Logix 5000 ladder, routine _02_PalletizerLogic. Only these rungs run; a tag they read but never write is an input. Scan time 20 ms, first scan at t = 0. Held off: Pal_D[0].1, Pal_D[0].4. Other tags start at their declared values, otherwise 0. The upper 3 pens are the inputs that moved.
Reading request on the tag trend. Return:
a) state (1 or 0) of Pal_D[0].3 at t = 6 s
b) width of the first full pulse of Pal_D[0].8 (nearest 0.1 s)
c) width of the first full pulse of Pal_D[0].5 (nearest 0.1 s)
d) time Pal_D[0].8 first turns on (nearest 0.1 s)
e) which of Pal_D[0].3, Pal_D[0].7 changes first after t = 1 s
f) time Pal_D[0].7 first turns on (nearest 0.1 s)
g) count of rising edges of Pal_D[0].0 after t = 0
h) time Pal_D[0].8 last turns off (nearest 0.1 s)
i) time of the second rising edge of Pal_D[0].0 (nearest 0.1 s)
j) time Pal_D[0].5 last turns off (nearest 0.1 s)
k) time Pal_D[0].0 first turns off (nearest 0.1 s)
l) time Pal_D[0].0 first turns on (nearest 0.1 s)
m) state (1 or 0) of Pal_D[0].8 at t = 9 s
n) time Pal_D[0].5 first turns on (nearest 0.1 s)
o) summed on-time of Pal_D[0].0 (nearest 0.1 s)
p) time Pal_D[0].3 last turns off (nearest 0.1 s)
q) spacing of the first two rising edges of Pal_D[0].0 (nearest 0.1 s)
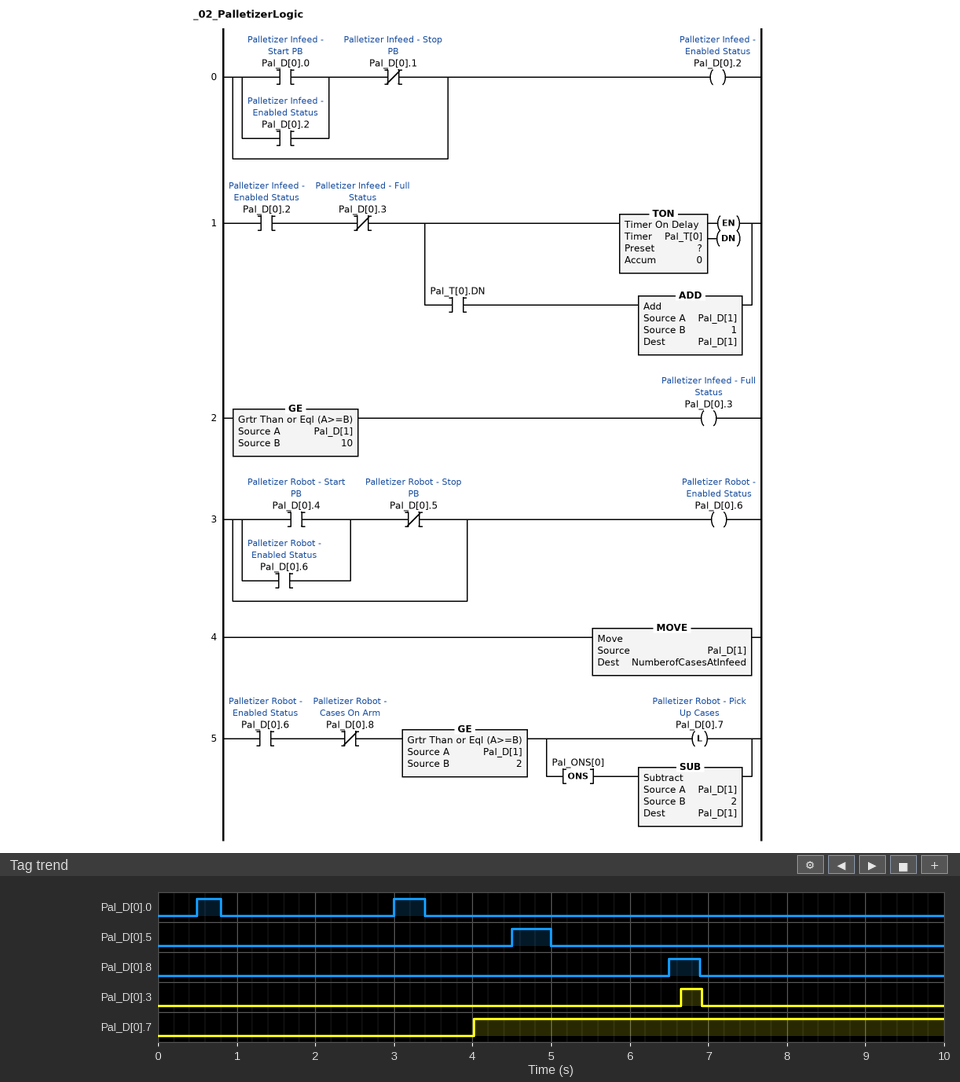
0
0.4 s
0.5 s
6.5 s
Pal_D[0].7
4.0 s
2
6.9 s
3.0 s
5.0 s
0.8 s
0.5 s
0
4.5 s
0.7 s
6.9 s
2.5 s
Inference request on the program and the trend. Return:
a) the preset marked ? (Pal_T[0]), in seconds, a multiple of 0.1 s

4.0 s
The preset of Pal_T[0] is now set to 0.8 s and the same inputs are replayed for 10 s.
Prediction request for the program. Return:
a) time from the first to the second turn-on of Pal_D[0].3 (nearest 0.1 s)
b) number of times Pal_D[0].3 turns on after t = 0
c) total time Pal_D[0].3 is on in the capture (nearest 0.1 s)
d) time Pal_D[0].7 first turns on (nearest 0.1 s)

1.1 s
2
2.5 s
0.8 s
